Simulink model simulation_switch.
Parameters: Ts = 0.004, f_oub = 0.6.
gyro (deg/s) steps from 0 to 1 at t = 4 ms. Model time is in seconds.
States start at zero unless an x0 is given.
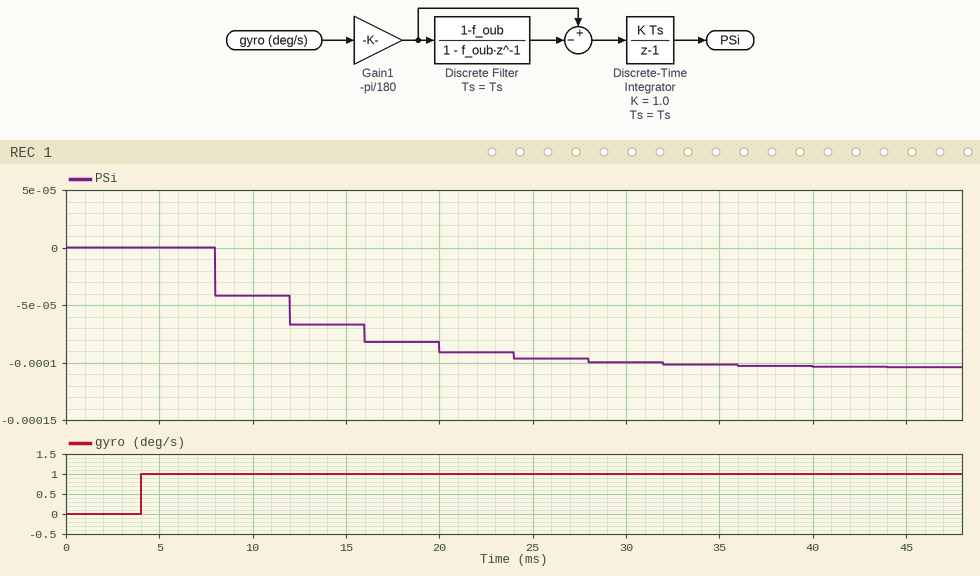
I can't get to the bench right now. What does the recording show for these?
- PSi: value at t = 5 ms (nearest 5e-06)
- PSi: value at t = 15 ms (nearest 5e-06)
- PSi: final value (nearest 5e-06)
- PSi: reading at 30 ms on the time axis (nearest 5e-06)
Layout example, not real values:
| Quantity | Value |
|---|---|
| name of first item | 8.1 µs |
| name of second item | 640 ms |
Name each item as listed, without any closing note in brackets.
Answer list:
| Quantity | Value |
|---|---|
| PSi: value at t = 5 ms | 0.000000 |
| PSi: value at t = 15 ms | -0.000065 |
| PSi: final value | -0.000105 |
| PSi: reading at 30 ms on the time axis | -0.000100 |
